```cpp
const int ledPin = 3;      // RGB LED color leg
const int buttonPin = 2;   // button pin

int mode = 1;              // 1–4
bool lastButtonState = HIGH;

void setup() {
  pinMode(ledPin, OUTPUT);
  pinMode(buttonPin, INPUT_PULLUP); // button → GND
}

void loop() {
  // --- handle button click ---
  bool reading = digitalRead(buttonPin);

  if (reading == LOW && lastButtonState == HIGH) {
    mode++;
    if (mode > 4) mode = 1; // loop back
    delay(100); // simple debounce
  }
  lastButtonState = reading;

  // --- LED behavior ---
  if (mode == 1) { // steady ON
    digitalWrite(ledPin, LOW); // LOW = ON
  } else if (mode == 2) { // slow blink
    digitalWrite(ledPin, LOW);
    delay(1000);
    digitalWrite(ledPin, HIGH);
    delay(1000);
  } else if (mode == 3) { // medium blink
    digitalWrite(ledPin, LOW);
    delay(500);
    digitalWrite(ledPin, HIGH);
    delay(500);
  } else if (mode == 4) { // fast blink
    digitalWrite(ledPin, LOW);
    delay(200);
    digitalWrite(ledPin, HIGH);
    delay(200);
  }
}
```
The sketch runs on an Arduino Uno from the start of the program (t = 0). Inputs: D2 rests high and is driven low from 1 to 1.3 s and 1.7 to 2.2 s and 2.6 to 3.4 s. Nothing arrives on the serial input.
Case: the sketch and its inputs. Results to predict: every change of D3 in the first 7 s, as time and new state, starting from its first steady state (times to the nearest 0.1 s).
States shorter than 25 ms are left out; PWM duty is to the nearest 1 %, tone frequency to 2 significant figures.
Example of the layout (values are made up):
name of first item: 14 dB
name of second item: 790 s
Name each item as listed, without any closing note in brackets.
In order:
every change of D3 in the first 7 s, as time and new state, starting from its first steady state: 0 s low; 2.1 s high; 3.1 s low; 4.1 s high; 5.1 s low; 6.1 s high
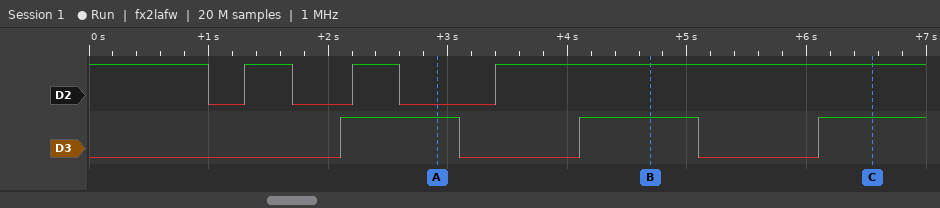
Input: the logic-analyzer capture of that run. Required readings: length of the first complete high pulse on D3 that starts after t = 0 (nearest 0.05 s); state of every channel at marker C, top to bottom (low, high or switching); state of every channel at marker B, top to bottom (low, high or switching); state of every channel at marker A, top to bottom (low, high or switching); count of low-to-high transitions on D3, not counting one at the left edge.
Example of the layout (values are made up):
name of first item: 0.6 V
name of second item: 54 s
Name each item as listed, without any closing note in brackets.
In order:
length of the first complete high pulse on D3 that starts after t = 0: 1.00 s
state of every channel at marker C, top to bottom: D2 high, D3 high
state of every channel at marker B, top to bottom: D2 high, D3 high
state of every channel at marker A, top to bottom: D2 low, D3 high
count of low-to-high transitions on D3, not counting one at the left edge: 3
